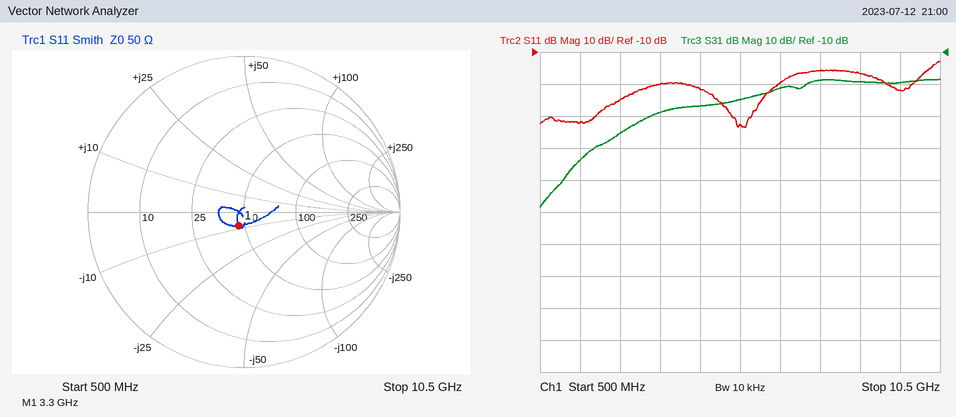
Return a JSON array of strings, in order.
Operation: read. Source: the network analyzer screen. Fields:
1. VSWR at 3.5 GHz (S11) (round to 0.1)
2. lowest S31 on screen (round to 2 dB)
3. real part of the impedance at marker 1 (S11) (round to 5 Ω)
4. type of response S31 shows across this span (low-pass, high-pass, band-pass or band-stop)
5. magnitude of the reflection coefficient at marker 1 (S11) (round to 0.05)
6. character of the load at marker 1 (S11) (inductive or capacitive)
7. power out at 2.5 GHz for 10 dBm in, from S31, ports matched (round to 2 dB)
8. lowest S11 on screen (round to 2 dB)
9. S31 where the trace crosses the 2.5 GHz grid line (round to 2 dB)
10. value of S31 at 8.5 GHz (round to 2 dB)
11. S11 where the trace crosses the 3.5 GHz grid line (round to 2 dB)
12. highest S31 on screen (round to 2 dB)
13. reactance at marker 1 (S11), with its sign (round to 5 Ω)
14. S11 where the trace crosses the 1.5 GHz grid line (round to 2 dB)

["1.2", "-58 dB", "45 Ω", "high-pass", "0.10", "capacitive", "-26 dBm", "-34 dB", "-36 dB", "-20 dB", "-20 dB", "-18 dB", "-10 Ω", "-32 dB"]
